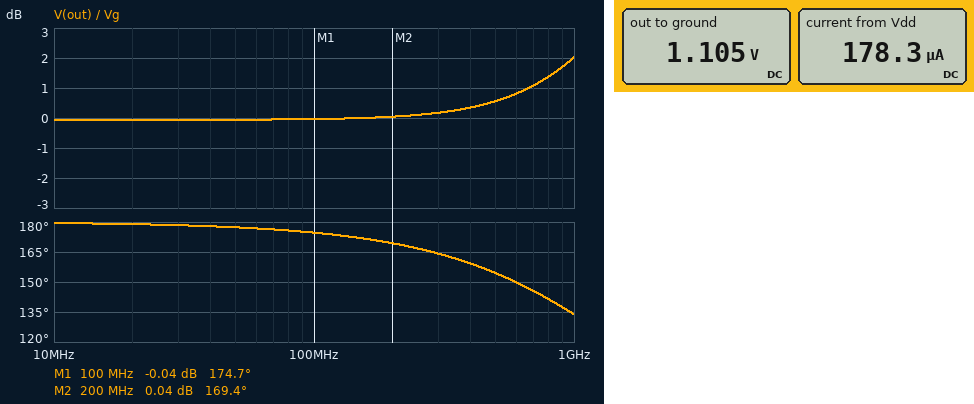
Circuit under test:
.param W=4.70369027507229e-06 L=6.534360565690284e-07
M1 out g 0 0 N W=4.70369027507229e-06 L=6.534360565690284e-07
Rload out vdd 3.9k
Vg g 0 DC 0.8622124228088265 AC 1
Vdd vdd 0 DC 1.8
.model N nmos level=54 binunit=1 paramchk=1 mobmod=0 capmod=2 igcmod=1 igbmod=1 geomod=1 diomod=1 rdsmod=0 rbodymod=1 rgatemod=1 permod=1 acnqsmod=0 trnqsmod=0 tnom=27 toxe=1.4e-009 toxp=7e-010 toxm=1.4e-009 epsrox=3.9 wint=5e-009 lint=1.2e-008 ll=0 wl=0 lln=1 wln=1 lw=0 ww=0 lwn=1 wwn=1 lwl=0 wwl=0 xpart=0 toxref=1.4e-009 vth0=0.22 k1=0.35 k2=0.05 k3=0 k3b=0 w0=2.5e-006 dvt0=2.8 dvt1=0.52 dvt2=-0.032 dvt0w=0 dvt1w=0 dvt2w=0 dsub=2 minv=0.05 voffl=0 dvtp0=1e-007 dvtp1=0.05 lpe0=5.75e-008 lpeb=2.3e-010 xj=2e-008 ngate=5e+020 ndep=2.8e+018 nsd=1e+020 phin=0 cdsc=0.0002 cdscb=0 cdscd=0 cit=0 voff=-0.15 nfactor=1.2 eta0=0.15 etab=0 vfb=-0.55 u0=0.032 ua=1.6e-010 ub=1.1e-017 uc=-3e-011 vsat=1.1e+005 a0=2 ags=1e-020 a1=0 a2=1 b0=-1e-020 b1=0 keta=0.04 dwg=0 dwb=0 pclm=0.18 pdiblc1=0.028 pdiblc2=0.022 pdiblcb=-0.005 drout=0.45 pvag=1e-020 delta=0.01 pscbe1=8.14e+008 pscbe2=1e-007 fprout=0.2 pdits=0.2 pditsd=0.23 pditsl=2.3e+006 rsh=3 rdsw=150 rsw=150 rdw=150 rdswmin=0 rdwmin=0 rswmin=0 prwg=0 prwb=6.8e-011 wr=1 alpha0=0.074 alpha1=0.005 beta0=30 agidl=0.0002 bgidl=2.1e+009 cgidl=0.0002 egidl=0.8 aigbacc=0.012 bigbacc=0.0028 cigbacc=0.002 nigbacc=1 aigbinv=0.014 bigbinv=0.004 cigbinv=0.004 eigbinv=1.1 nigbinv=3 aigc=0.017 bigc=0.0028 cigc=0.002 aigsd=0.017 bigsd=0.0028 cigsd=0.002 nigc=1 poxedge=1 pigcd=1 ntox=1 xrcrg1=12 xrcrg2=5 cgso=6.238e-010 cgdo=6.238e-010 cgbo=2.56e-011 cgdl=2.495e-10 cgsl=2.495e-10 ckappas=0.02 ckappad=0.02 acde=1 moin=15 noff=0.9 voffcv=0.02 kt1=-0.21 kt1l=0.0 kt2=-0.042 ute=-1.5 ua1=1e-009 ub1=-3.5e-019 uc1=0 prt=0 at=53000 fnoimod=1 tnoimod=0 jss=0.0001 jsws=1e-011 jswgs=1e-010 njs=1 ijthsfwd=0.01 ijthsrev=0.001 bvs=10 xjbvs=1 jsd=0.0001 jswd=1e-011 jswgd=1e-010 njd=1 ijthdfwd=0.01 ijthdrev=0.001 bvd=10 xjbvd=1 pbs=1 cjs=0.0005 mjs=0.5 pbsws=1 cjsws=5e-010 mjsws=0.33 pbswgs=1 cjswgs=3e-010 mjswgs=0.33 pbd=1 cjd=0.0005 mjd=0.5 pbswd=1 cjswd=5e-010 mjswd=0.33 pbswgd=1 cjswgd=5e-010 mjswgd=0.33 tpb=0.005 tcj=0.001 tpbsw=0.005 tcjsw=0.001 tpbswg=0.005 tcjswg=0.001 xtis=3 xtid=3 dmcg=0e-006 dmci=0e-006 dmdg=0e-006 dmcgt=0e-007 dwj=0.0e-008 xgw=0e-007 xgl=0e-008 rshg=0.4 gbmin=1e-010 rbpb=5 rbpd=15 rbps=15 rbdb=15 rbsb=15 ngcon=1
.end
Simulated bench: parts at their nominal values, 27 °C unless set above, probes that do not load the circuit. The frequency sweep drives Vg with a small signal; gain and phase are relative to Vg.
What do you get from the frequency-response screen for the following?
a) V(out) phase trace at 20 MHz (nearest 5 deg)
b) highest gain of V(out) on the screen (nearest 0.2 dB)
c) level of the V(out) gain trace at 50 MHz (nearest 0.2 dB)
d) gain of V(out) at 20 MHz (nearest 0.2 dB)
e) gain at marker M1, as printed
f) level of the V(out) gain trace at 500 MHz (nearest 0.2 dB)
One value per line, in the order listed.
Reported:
180 deg
2.0 dB
0 dB
0 dB
-0.04 dB
0.6 dB
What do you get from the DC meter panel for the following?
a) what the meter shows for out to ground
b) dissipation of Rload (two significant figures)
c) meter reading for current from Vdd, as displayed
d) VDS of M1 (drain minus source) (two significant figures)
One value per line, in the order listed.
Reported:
1.105 V
120 µW
178.3 µA
1.1 V
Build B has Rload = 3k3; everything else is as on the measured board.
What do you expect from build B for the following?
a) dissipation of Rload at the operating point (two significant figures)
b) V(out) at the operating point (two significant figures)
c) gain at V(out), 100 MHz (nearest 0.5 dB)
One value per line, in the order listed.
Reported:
110 µW
1.2 V
-1.5 dB
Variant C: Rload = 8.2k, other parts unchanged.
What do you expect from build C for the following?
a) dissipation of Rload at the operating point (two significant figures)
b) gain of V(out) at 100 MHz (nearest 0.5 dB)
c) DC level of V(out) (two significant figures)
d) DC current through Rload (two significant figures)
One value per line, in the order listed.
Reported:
220 µW
2.5 dB
460 mV
160 µA
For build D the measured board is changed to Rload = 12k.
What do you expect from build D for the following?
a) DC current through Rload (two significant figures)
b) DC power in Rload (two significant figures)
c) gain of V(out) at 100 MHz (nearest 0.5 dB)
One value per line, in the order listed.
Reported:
130 µA
200 µW
-11.0 dB
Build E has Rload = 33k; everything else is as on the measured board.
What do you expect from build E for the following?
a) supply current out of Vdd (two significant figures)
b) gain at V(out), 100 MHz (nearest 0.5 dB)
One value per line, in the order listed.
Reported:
52 µA
-23.0 dB
